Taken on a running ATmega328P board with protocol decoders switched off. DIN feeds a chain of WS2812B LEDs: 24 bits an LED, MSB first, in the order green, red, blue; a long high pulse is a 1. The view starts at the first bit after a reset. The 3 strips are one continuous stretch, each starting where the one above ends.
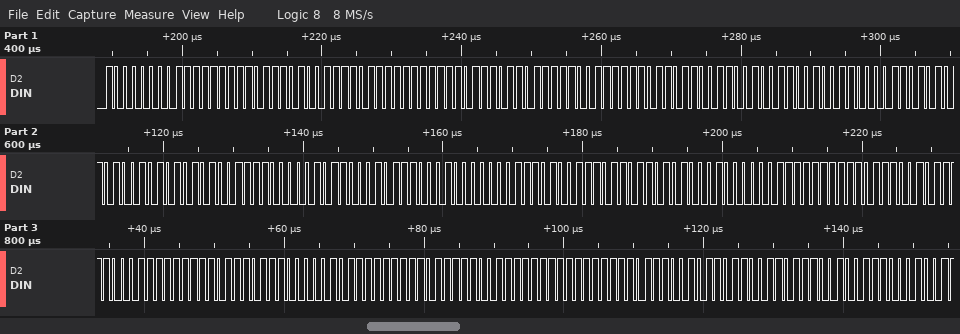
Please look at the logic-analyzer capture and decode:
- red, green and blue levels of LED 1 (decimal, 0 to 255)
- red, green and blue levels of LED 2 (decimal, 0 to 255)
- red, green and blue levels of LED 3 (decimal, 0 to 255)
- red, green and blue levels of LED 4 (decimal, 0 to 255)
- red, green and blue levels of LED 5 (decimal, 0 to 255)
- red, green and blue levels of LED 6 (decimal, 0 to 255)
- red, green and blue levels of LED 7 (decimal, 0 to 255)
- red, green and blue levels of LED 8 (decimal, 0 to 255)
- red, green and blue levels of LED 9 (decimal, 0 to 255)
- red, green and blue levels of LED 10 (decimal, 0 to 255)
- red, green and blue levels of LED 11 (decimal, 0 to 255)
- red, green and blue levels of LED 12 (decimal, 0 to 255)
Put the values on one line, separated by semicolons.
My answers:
255, 128, 186; 255, 123, 187; 253, 124, 179; 76, 38, 53; 170, 82, 120; 92, 44, 64; 237, 116, 168; 255, 129, 185; 255, 120, 187; 255, 130, 190; 255, 127, 185; 220, 108, 156
